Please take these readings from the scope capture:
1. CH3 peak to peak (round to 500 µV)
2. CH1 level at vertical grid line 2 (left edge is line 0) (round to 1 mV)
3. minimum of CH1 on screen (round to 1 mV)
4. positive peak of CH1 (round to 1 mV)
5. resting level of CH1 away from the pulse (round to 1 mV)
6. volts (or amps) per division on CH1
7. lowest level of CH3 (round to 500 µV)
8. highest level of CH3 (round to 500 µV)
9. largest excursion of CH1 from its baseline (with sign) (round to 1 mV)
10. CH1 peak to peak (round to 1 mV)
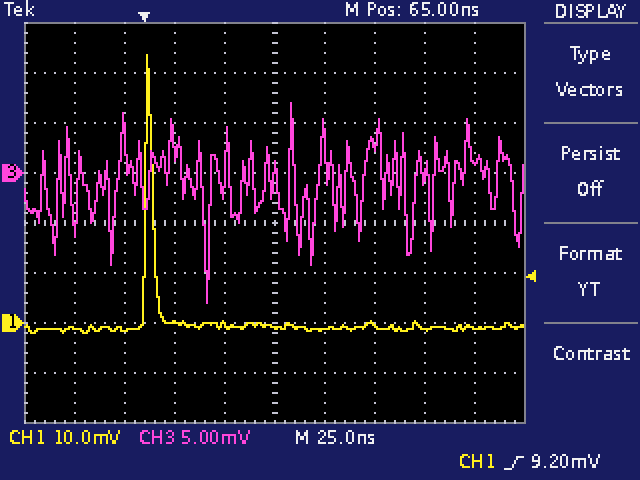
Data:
20.0 mV
-1 mV
-2 mV
54 mV
-1 mV
10 mV
-13.0 mV
7.0 mV
+55 mV
56 mV
